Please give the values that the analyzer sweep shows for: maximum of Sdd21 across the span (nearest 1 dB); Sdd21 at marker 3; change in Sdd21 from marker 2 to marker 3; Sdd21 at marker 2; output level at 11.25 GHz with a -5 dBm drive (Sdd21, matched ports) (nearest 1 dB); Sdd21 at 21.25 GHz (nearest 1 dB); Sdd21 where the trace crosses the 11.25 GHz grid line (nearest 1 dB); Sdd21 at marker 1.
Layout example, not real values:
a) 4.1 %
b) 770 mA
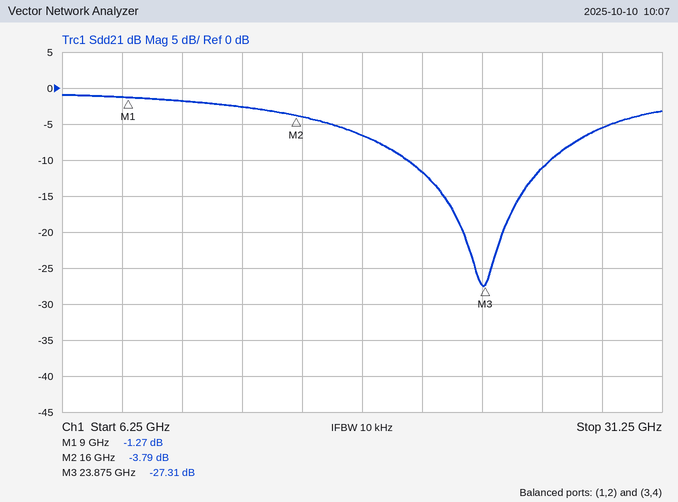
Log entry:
a) -1 dB
b) -27.31 dB
c) -23.52 dB
d) -3.79 dB
e) -7 dBm
f) -12 dB
g) -2 dB
h) -1.27 dB
